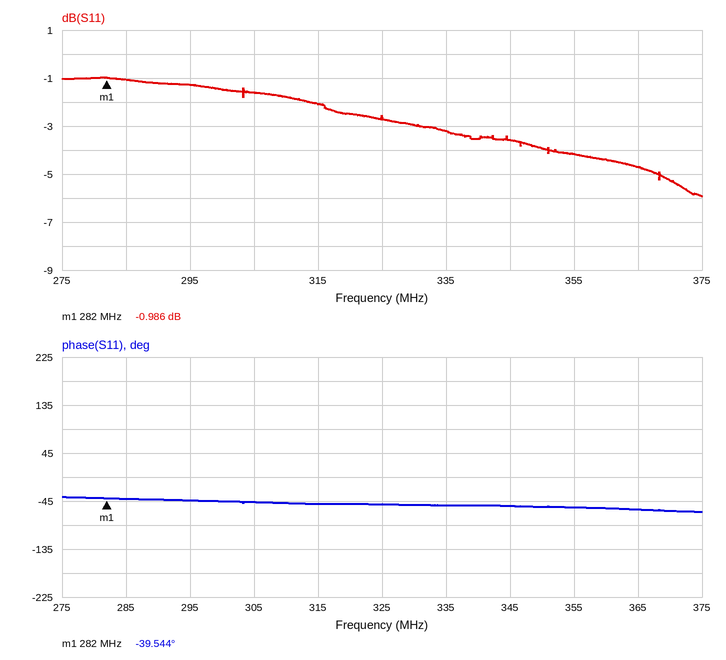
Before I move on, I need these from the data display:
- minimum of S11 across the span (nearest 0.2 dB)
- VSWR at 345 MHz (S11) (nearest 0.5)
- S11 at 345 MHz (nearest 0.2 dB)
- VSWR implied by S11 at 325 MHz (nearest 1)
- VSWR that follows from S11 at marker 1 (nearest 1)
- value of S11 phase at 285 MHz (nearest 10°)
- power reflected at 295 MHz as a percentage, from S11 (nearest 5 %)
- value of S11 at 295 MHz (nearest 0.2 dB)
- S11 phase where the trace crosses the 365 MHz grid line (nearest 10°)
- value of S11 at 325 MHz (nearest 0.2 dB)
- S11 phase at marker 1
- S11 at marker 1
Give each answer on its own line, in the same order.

-6.0 dB
5.0
-3.6 dB
7
18
-40°
75 %
-1.2 dB
-60°
-2.6 dB
-39.544°
-0.986 dB
